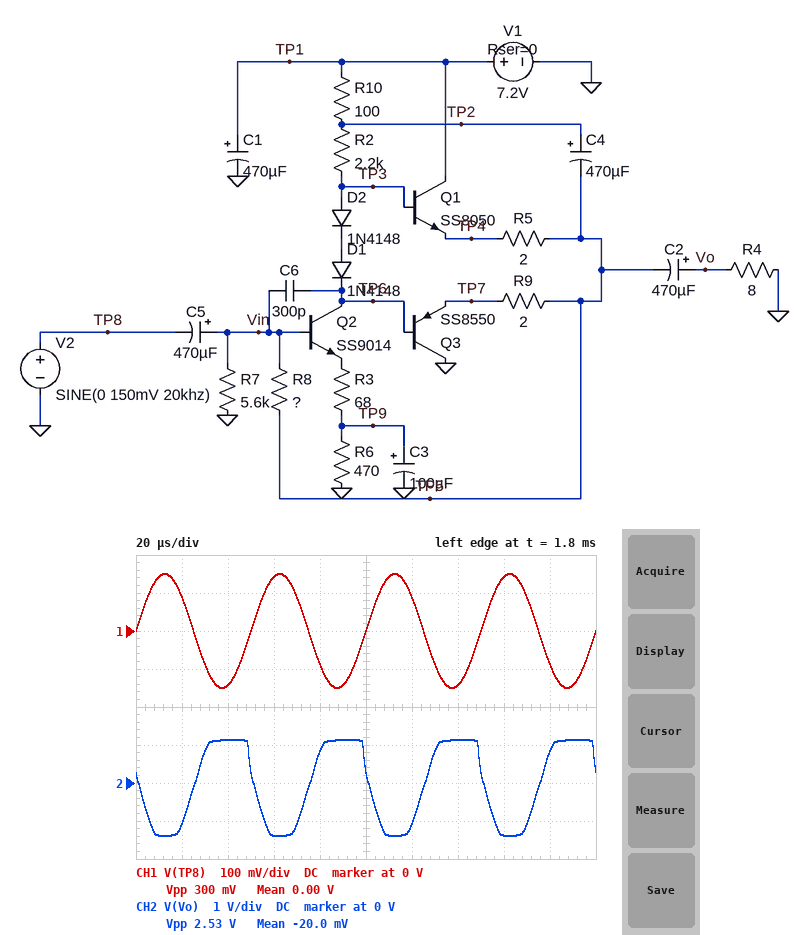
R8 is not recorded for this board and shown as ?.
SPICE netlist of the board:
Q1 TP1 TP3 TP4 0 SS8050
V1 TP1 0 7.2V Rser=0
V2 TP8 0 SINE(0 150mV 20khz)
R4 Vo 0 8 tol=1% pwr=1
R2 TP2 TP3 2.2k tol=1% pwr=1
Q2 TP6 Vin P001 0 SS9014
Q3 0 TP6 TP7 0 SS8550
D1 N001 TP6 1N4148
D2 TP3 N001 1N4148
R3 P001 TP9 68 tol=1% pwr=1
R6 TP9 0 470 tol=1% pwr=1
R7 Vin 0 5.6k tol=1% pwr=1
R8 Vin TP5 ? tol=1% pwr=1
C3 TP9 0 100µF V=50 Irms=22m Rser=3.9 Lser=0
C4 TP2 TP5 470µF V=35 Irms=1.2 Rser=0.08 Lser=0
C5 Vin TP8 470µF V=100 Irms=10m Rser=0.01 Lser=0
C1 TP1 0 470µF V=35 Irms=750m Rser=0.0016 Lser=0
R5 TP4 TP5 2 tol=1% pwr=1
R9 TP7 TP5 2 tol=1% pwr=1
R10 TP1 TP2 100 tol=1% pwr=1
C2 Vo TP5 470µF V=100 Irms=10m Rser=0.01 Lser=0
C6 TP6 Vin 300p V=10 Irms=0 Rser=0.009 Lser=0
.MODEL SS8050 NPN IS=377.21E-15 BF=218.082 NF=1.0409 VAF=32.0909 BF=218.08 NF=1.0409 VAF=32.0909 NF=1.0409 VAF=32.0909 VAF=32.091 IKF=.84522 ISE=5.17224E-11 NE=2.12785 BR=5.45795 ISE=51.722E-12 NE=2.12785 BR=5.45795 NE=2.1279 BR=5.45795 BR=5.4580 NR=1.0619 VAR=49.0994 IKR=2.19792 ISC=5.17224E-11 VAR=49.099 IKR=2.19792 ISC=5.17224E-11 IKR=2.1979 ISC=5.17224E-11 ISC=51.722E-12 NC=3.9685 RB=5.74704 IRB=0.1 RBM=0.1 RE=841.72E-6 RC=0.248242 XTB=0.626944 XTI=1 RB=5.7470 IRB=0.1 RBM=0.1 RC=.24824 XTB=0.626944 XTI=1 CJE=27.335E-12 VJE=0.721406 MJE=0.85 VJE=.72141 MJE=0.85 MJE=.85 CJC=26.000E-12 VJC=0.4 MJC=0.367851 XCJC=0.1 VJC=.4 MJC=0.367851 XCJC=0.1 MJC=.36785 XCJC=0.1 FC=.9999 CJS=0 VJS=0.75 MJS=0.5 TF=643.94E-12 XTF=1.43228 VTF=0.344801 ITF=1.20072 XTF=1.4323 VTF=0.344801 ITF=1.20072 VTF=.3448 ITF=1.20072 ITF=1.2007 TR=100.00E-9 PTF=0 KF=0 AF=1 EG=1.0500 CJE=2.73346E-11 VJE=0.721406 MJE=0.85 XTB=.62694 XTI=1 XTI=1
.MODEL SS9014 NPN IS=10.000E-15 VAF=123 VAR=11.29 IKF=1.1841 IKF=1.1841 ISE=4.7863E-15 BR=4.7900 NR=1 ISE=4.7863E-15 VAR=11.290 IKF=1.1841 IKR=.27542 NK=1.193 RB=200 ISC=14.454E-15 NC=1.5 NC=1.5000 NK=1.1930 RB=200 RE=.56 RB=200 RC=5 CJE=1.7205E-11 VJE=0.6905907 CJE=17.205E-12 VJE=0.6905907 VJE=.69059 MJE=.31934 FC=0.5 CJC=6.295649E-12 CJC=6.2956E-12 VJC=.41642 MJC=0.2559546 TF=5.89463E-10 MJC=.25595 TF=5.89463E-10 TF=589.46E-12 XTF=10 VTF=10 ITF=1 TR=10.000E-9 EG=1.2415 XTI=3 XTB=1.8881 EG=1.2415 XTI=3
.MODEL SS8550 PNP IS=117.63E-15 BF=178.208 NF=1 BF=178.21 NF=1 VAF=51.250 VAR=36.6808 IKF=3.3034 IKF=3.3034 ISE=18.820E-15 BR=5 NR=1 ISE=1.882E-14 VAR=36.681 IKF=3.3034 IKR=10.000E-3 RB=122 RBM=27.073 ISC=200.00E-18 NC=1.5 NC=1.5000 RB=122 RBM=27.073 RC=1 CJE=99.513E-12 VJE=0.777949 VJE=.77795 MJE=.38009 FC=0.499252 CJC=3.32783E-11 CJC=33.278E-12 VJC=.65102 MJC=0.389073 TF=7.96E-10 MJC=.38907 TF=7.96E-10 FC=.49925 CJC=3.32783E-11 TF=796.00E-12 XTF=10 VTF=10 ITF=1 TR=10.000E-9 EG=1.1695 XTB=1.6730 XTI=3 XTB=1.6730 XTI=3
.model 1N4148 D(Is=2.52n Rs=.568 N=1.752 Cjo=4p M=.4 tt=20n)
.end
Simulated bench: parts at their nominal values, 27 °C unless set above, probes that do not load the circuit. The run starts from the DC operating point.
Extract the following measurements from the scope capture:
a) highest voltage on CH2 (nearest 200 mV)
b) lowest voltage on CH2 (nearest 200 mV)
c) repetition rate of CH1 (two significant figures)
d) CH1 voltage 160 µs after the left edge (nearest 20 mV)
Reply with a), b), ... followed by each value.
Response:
a) 1.2 V
b) -1.4 V
c) 20 kHz
d) 140 mV
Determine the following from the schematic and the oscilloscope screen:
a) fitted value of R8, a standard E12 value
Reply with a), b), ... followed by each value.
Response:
a) 8.2 kΩ
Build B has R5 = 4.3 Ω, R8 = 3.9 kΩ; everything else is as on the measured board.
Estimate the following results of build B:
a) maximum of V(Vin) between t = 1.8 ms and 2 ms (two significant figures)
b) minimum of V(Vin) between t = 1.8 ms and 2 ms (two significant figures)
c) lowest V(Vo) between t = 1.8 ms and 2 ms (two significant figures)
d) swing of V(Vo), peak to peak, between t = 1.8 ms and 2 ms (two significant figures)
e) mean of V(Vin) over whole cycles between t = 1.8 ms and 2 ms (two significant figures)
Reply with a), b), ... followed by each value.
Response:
a) 1.7 V
b) 1.4 V
c) -790 mV
d) 1.9 V
e) 1.6 V
